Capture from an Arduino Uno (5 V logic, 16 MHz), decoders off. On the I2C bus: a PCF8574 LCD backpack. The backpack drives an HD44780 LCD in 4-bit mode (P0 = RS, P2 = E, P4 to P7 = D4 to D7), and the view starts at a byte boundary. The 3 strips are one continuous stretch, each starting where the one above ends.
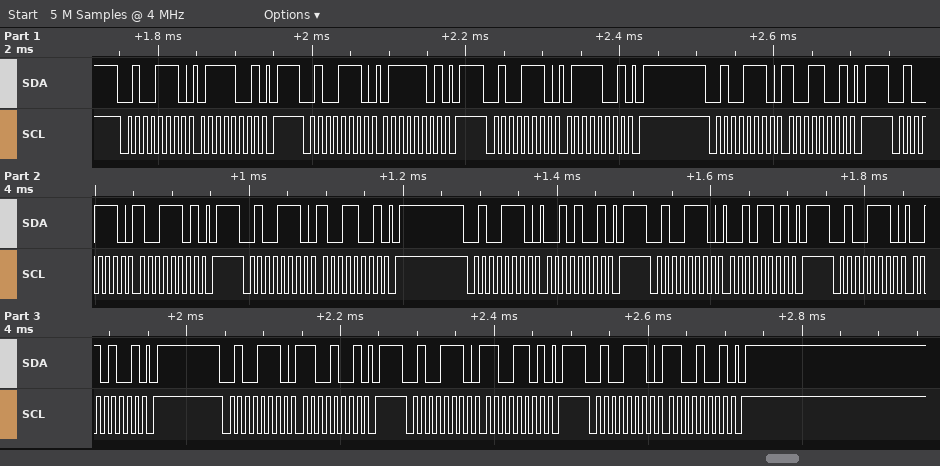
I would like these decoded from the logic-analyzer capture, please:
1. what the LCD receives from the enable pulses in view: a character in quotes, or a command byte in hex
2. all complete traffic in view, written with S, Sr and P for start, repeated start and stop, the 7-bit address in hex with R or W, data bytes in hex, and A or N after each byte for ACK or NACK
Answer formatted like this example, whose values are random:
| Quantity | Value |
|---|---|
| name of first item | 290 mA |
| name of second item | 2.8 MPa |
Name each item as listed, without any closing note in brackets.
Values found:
| Quantity | Value |
|---|---|
| what the LCD receives from the enable pulses in view: a character in quotes, or a command byte in hex | 'y' ',' |
| all complete traffic in view, written with S, Sr and P for start, repeated start and stop, the 7-bit address in hex with R or W, data bytes in hex, and A or N after each byte for ACK or NACK | S 27W A 79 A P S 27W A 7D A P S 27W A 79 A P S 27W A 99 A P S 27W A 9D A P S 27W A 99 A P S 27W A 29 A P S 27W A 2D A P S 27W A 29 A P S 27W A C9 A P S 27W A CD A P S 27W A C9 A P |
